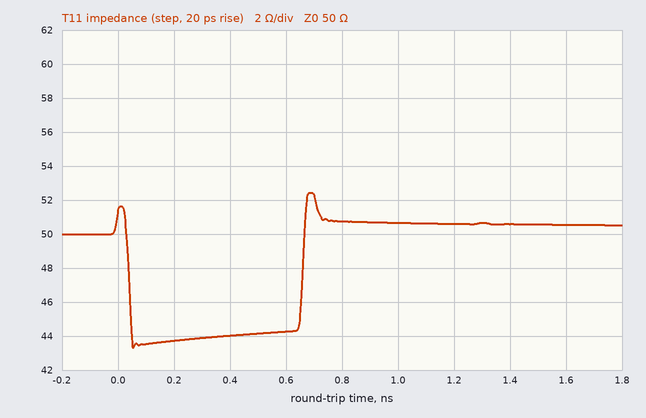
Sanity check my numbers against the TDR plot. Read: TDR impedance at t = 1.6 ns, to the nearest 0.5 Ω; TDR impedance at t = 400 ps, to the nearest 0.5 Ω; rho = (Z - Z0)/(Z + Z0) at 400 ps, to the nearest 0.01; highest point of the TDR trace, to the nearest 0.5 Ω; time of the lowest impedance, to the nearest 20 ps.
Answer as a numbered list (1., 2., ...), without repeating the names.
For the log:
1. 50.5 Ω
2. 44.0 Ω
3. -0.06
4. 52.5 Ω
5. 60 ps
